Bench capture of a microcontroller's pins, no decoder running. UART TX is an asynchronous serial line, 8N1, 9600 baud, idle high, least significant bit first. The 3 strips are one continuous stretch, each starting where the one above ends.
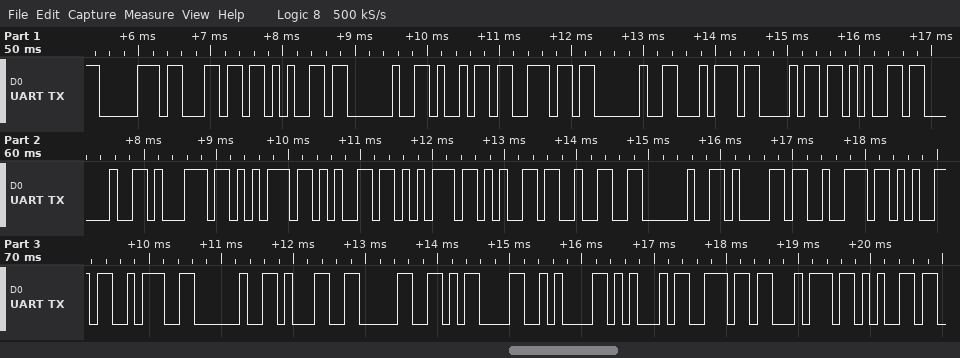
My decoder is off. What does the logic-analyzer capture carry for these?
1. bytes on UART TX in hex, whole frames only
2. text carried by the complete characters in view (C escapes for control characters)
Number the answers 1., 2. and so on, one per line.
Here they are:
1. 70 6C 65 20 69 6E 20 74 68 65 20 71 75 65 75 65 32 20 61 72 65 3A 20 31 30 0D 0A 45 6E 74 65
2. "ple in the queue2 are: 10\r\nEnte"
